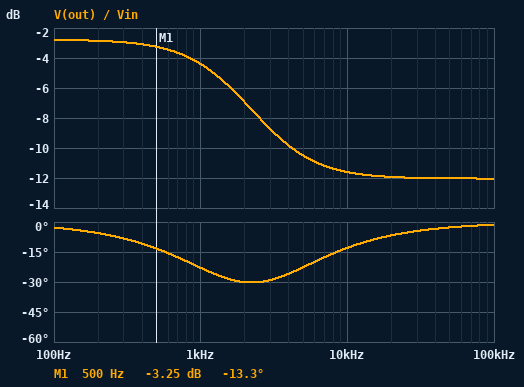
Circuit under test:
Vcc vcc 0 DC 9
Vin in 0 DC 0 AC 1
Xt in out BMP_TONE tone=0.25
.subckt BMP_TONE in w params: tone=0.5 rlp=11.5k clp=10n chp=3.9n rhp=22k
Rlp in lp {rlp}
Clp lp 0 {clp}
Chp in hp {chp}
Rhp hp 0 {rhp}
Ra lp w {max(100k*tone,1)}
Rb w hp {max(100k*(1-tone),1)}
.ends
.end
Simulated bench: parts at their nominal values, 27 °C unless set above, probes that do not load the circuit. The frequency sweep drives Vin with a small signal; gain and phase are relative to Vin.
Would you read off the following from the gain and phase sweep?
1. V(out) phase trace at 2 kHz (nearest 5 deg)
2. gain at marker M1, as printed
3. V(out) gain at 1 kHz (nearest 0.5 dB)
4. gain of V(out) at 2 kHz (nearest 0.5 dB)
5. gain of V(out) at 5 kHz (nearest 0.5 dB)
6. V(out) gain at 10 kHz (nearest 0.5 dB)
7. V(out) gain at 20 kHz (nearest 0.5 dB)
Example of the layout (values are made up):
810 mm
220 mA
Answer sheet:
-30 deg
-3.25 dB
-4.5 dB
-7.0 dB
-10.5 dB
-11.5 dB
-12.0 dB
